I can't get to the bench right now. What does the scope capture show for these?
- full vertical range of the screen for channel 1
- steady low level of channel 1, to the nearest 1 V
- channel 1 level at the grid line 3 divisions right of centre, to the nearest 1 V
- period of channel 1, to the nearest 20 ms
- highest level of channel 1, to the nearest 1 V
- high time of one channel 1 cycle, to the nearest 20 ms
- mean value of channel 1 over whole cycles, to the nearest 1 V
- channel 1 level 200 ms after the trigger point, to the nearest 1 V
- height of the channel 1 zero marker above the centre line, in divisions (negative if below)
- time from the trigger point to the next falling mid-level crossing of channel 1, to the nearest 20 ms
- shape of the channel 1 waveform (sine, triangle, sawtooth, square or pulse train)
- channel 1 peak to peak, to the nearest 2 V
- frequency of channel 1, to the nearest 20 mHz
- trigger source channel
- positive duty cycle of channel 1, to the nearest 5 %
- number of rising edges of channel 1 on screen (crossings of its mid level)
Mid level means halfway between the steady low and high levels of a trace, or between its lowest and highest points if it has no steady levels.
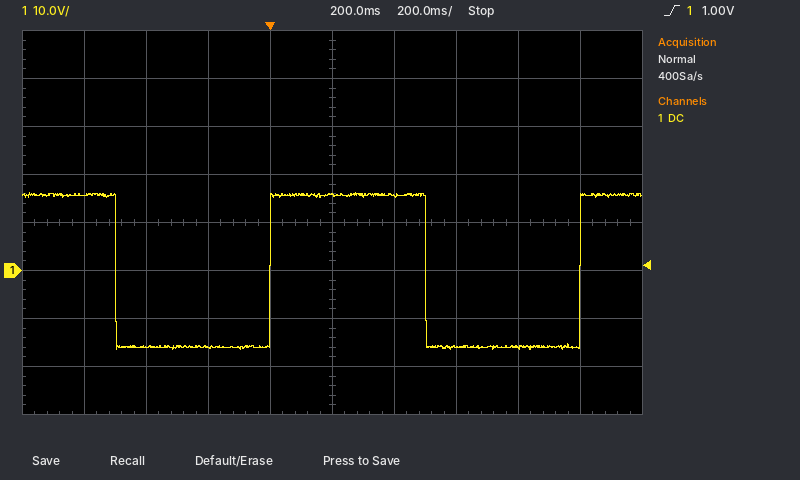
80 V
-16 V
-16 V
1.00 s
16 V
500 ms
0 V
16 V
-1.0 div
500 ms
square
32 V
1.00 Hz
channel 1
50 %
2
